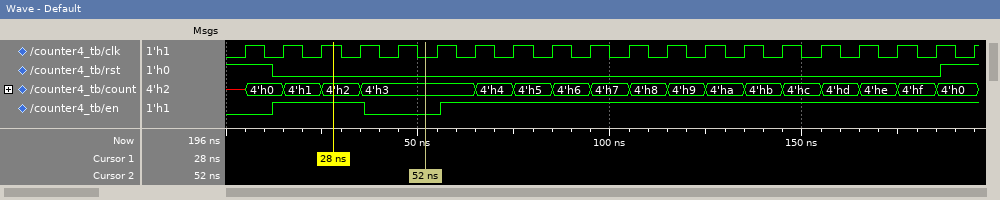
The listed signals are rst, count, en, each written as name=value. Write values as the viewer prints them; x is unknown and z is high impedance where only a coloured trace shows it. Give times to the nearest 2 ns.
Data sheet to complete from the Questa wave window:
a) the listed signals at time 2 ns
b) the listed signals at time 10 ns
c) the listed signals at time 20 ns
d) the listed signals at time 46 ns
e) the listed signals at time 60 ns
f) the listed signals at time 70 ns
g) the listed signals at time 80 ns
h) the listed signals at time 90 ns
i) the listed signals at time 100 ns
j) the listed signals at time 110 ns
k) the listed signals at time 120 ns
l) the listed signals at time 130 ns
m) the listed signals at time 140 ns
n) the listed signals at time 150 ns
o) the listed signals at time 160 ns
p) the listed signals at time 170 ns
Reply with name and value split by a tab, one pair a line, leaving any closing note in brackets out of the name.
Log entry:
the listed signals at time 2 ns	rst=1, count=x, en=0
the listed signals at time 10 ns	rst=1, count=4'h0, en=0
the listed signals at time 20 ns	rst=0, count=4'h1, en=1
the listed signals at time 46 ns	rst=0, count=4'h3, en=0
the listed signals at time 60 ns	rst=0, count=4'h3, en=1
the listed signals at time 70 ns	rst=0, count=4'h4, en=1
the listed signals at time 80 ns	rst=0, count=4'h5, en=1
the listed signals at time 90 ns	rst=0, count=4'h6, en=1
the listed signals at time 100 ns	rst=0, count=4'h7, en=1
the listed signals at time 110 ns	rst=0, count=4'h8, en=1
the listed signals at time 120 ns	rst=0, count=4'h9, en=1
the listed signals at time 130 ns	rst=0, count=4'ha, en=1
the listed signals at time 140 ns	rst=0, count=4'hb, en=1
the listed signals at time 150 ns	rst=0, count=4'hc, en=1
the listed signals at time 160 ns	rst=0, count=4'hd, en=1
the listed signals at time 170 ns	rst=0, count=4'he, en=1
